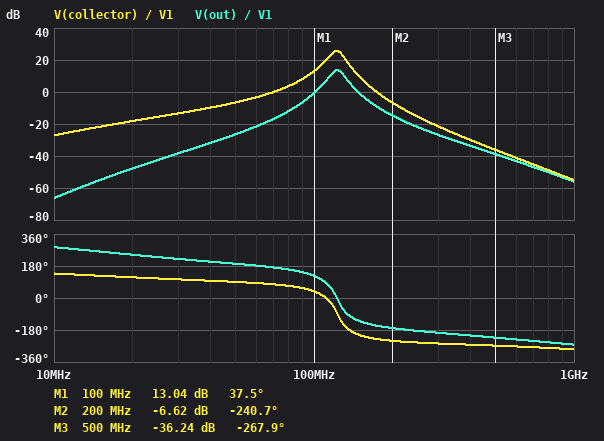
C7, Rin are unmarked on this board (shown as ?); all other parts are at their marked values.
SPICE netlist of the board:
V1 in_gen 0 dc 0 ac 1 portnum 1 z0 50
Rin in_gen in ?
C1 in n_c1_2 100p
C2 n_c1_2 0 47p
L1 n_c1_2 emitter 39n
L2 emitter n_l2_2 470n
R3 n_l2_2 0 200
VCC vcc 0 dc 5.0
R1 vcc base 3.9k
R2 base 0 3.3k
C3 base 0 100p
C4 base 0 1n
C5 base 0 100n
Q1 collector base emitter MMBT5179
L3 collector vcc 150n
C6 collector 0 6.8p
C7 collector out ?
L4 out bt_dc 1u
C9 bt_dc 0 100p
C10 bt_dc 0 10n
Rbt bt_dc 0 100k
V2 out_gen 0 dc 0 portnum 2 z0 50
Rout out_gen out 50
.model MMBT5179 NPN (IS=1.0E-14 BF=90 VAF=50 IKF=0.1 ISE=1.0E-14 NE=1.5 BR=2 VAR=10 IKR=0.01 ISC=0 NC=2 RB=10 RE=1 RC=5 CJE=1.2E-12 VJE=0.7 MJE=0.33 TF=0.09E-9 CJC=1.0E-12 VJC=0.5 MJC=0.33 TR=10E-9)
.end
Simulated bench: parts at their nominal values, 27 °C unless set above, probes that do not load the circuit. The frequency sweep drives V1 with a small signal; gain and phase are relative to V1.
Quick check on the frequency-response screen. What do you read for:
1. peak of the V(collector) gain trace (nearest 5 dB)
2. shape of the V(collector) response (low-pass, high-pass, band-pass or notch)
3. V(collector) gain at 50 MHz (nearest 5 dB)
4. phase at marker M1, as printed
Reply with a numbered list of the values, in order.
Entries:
1. 25 dB
2. band-pass
3. -5 dB
4. 37.5 deg
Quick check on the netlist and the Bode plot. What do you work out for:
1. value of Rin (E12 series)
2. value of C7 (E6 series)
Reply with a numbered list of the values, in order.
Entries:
1. 82 Ω
2. 3.3 pF
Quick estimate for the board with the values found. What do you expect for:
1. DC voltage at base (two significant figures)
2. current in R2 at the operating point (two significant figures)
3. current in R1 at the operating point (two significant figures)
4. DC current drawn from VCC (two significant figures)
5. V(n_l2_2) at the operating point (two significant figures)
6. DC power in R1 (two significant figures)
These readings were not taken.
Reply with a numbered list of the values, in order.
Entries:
1. 2.1 V
2. 650 µA
3. 730 µA
4. 7.8 mA
5. 1.4 V
6. 2.1 mW
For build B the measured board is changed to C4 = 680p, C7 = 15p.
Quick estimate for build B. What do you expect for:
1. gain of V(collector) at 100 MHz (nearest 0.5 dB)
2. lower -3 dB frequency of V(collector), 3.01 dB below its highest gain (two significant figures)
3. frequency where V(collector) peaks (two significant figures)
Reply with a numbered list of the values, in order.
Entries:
1. 9.5 dB
2. 84 MHz
3. 110 MHz
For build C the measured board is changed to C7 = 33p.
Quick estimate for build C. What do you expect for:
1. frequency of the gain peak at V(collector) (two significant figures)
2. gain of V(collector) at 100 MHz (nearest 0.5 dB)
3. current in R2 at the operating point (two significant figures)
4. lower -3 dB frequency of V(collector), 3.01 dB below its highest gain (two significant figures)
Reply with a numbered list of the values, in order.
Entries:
1. 110 MHz
2. 5.0 dB
3. 650 µA
4. 89 MHz
